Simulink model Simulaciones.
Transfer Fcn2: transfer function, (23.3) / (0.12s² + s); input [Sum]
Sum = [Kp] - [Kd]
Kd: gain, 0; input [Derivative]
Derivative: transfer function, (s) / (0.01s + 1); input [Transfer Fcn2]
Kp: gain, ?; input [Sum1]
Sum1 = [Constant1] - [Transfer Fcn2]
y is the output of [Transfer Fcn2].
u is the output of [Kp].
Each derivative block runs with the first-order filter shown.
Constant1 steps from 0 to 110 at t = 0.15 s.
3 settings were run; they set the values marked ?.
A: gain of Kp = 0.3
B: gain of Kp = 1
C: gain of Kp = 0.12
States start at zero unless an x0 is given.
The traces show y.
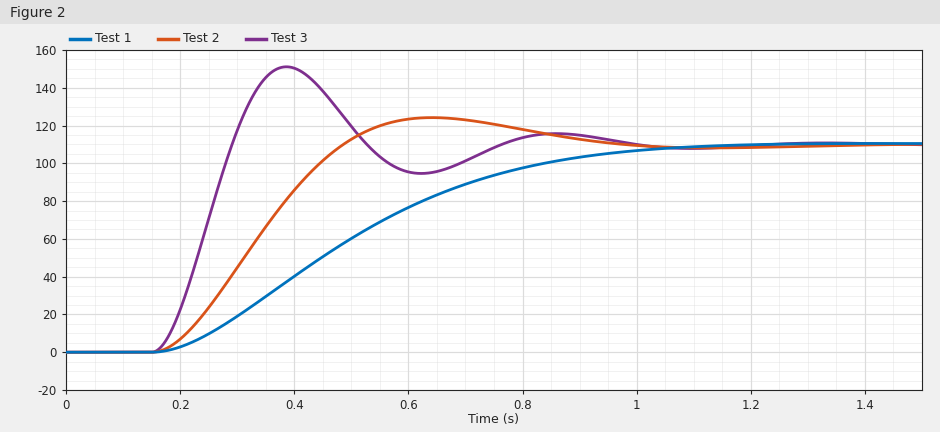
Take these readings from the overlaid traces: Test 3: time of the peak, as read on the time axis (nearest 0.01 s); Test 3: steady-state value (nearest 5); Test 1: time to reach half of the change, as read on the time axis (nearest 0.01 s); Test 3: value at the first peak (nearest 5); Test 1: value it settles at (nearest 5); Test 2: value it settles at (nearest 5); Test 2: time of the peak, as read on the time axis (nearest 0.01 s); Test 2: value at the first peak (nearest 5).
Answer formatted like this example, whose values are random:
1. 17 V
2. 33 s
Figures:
1. 0.39 s
2. 110
3. 0.47 s
4. 150
5. 110
6. 110
7. 0.64 s
8. 125
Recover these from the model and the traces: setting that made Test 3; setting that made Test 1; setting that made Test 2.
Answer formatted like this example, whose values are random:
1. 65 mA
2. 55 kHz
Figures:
1. B
2. C
3. A
